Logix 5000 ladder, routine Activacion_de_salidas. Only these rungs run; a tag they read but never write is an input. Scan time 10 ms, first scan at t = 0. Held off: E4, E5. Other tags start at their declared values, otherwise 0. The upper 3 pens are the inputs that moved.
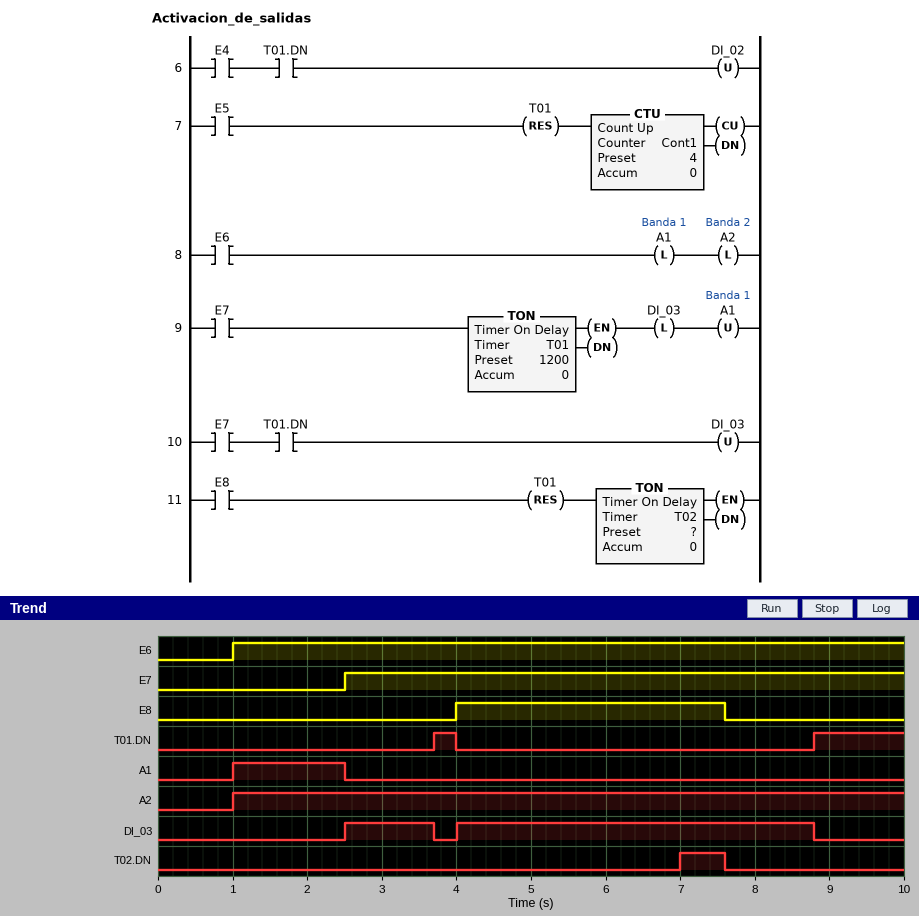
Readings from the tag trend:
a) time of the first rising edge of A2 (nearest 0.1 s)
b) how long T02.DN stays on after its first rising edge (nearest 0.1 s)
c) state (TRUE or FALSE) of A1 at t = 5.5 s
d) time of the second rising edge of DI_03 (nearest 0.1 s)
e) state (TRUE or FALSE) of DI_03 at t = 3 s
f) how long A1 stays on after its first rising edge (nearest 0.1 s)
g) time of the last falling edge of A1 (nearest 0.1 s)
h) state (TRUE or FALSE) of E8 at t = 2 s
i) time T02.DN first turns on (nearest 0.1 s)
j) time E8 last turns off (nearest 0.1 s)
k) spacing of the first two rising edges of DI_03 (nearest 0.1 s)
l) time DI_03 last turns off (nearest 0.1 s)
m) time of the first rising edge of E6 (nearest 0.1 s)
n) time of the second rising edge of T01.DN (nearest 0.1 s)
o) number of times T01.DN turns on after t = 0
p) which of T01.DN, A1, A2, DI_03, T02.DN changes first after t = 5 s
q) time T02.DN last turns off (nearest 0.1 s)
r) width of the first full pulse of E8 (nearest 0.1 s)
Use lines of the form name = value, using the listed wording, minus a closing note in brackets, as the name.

time of the first rising edge of A2 = 1.0 s
how long T02.DN stays on after its first rising edge = 0.6 s
state (TRUE or FALSE) of A1 at t = 5.5 s = FALSE
time of the second rising edge of DI_03 = 4.0 s
state (TRUE or FALSE) of DI_03 at t = 3 s = TRUE
how long A1 stays on after its first rising edge = 1.5 s
time of the last falling edge of A1 = 2.5 s
state (TRUE or FALSE) of E8 at t = 2 s = FALSE
time T02.DN first turns on = 7.0 s
time E8 last turns off = 7.6 s
spacing of the first two rising edges of DI_03 = 1.5 s
time DI_03 last turns off = 8.8 s
time of the first rising edge of E6 = 1.0 s
time of the second rising edge of T01.DN = 8.8 s
number of times T01.DN turns on after t = 0 = 2
which of T01.DN, A1, A2, DI_03, T02.DN changes first after t = 5 s = T02.DN
time T02.DN last turns off = 7.6 s
width of the first full pulse of E8 = 3.6 s
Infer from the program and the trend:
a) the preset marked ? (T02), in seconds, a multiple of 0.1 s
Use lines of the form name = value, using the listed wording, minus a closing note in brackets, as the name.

the preset marked ? (T02), in seconds, a multiple of 0.1 s = 3.0 s
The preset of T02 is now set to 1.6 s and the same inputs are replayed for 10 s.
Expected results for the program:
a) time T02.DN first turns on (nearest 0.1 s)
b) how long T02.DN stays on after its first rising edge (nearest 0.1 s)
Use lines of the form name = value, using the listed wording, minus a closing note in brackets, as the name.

time T02.DN first turns on = 5.6 s
how long T02.DN stays on after its first rising edge = 2.0 s
